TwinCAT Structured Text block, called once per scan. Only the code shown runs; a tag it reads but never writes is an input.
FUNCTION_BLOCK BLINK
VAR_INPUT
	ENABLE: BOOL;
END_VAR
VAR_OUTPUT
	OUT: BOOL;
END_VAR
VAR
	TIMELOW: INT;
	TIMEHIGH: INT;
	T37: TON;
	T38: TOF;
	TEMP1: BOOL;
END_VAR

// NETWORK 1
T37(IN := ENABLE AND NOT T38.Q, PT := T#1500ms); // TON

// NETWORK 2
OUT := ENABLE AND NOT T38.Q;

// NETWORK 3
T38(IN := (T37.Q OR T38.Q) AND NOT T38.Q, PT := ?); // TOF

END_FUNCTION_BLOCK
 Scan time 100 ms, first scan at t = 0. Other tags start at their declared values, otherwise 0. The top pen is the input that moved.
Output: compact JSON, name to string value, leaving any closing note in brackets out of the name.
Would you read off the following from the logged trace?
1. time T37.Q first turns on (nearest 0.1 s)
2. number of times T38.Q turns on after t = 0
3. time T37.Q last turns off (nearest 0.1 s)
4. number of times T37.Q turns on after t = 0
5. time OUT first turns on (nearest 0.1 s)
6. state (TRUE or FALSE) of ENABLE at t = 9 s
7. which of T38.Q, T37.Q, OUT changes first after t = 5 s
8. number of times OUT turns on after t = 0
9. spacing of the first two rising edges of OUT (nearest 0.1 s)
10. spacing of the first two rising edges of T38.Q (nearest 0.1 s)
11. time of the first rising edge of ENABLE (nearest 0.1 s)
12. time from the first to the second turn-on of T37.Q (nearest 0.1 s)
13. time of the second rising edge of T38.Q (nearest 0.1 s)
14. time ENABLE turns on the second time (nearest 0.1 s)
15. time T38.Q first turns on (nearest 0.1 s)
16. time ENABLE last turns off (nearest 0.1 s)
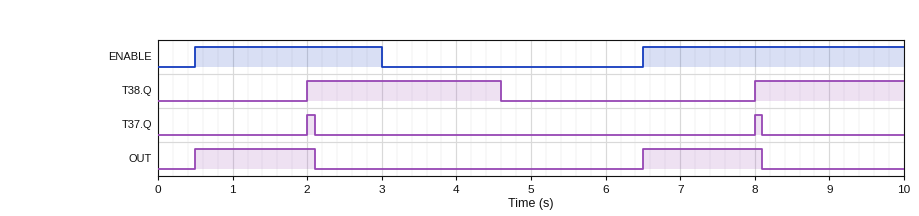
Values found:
{"time T37.Q first turns on": "2.0 s", "number of times T38.Q turns on after t = 0": "2", "time T37.Q last turns off": "8.1 s", "number of times T37.Q turns on after t = 0": "2", "time OUT first turns on": "0.5 s", "state (TRUE or FALSE) of ENABLE at t = 9 s": "TRUE", "which of T38.Q, T37.Q, OUT changes first after t = 5 s": "OUT", "number of times OUT turns on after t = 0": "2", "spacing of the first two rising edges of OUT": "6.0 s", "spacing of the first two rising edges of T38.Q": "6.0 s", "time of the first rising edge of ENABLE": "0.5 s", "time from the first to the second turn-on of T37.Q": "6.0 s", "time of the second rising edge of T38.Q": "8.0 s", "time ENABLE turns on the second time": "6.5 s", "time T38.Q first turns on": "2.0 s", "time ENABLE last turns off": "3.0 s"}
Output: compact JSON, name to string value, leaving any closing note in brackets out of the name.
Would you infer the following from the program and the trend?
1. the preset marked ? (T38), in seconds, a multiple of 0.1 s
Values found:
{"the preset marked ? (T38), in seconds, a multiple of 0.1 s": "2.5 s"}
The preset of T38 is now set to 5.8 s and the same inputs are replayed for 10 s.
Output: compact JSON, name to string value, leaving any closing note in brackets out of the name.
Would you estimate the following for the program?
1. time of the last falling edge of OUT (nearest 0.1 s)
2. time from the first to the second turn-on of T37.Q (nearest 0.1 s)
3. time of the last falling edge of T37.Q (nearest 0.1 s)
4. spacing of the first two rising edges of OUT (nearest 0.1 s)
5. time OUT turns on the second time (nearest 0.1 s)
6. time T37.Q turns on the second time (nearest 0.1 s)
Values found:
{"time of the last falling edge of OUT": "9.6 s", "time from the first to the second turn-on of T37.Q": "7.5 s", "time of the last falling edge of T37.Q": "9.6 s", "spacing of the first two rising edges of OUT": "7.5 s", "time OUT turns on the second time": "8.0 s", "time T37.Q turns on the second time": "9.5 s"}
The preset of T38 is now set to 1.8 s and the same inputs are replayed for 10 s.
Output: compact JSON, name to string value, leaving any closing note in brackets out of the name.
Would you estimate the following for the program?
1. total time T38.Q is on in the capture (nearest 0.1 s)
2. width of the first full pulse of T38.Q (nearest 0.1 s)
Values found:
{"total time T38.Q is on in the capture": "3.8 s", "width of the first full pulse of T38.Q": "1.9 s"}
